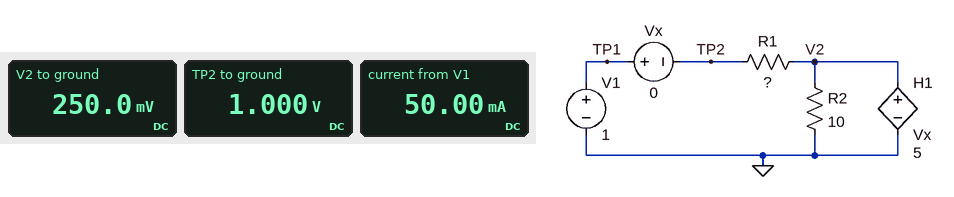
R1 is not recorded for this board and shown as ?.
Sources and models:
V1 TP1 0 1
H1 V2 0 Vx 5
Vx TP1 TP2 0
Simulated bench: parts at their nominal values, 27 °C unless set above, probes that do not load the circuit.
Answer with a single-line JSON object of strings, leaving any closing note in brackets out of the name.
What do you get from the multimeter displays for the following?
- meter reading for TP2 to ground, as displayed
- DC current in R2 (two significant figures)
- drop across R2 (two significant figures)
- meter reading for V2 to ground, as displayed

{"meter reading for TP2 to ground, as displayed": "1.000 V", "DC current in R2": "25 mA", "drop across R2": "250 mV", "meter reading for V2 to ground, as displayed": "250.0 mV"}
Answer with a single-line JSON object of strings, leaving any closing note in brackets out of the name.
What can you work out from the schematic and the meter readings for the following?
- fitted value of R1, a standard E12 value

{"fitted value of R1, a standard E12 value": "15 Ω"}
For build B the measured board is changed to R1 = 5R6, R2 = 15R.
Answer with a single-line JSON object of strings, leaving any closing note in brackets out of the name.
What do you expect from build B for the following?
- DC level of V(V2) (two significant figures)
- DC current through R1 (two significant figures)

{"DC level of V(V2)": "470 mV", "DC current through R1": "94 mA"}
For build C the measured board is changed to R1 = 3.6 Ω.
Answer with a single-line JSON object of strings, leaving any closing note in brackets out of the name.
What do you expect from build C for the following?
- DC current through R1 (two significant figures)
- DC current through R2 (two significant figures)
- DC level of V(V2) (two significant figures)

{"DC current through R1": "120 mA", "DC current through R2": "58 mA", "DC level of V(V2)": "580 mV"}
